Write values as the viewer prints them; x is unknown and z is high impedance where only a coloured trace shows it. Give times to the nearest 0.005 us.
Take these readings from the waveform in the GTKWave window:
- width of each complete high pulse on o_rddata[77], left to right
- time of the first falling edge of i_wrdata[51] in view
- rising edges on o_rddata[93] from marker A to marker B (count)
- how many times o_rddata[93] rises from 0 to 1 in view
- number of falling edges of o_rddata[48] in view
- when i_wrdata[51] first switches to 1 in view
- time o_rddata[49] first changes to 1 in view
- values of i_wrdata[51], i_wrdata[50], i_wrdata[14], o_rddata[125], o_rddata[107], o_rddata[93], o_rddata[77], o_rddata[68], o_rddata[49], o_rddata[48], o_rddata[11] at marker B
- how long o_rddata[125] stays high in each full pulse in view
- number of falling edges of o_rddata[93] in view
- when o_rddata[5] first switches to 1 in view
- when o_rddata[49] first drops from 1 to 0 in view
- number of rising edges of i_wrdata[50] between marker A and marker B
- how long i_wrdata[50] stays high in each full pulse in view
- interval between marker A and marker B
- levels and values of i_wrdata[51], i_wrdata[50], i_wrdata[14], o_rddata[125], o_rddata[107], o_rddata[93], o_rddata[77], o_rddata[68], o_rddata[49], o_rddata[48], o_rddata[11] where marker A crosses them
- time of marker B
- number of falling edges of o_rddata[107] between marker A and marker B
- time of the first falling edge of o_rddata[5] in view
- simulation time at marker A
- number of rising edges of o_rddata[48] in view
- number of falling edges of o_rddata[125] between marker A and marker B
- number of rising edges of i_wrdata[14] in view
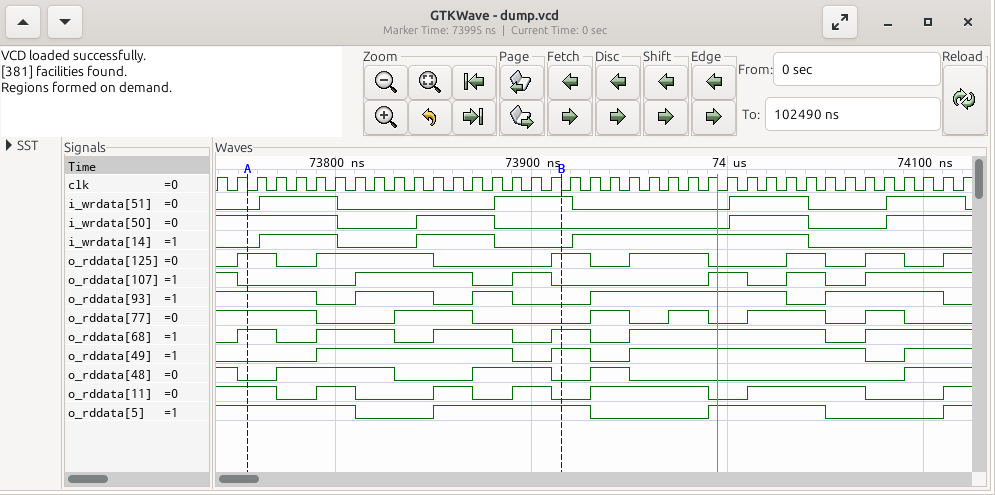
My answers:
0.04 us, 0.02 us, 0.02 us, 0.04 us, 0.02 us
73.8 us
2
4
4
73.76 us
73.79 us
i_wrdata[51]=1, i_wrdata[50]=0, i_wrdata[14]=0, o_rddata[125]=1, o_rddata[107]=0, o_rddata[93]=0, o_rddata[77]=0, o_rddata[68]=1, o_rddata[49]=1, o_rddata[48]=0, o_rddata[11]=0
0.02 us, 0.06 us, 0.02 us, 0.04 us, 0.02 us, 0.02 us
5
73.85 us
73.89 us
1
0.04 us, 0.04 us
0.16 us
i_wrdata[51]=0, i_wrdata[50]=1, i_wrdata[14]=0, o_rddata[125]=1, o_rddata[107]=0, o_rddata[93]=1, o_rddata[77]=1, o_rddata[68]=1, o_rddata[49]=0, o_rddata[48]=0, o_rddata[11]=1
73.915 us
2
73.81 us
73.755 us
4
2
3
